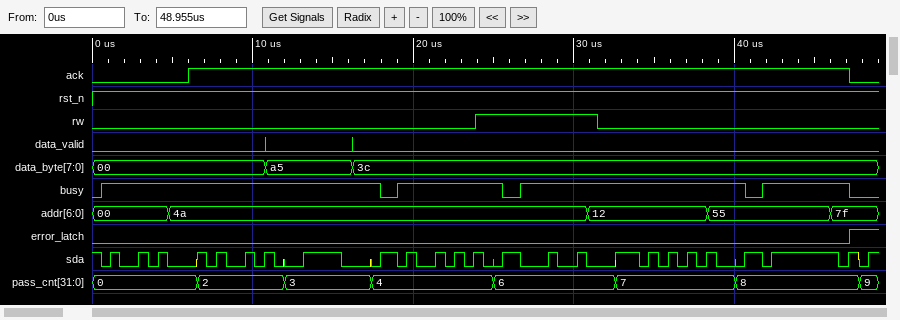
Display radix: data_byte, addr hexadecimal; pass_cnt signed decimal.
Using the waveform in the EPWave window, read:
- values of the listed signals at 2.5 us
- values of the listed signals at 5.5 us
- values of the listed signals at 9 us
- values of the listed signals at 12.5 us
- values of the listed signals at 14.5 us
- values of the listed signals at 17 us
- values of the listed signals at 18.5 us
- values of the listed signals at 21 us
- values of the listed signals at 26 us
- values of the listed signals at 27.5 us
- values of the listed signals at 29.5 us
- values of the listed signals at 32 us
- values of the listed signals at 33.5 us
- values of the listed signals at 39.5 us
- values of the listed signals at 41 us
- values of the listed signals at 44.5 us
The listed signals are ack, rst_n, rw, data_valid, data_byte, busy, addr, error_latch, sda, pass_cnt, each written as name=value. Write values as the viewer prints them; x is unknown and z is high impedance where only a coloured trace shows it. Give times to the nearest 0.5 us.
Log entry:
ack=0, rst_n=1, rw=0, data_valid=0, data_byte=00, busy=1, addr=00, error_latch=0, sda=0, pass_cnt=0
ack=0, rst_n=1, rw=0, data_valid=0, data_byte=00, busy=1, addr=4a, error_latch=0, sda=0, pass_cnt=0
ack=1, rst_n=1, rw=0, data_valid=0, data_byte=00, busy=1, addr=4a, error_latch=0, sda=0, pass_cnt=2
ack=1, rst_n=1, rw=0, data_valid=0, data_byte=a5, busy=1, addr=4a, error_latch=0, sda=0, pass_cnt=3
ack=1, rst_n=1, rw=0, data_valid=0, data_byte=a5, busy=1, addr=4a, error_latch=0, sda=1, pass_cnt=3
ack=1, rst_n=1, rw=0, data_valid=0, data_byte=3c, busy=1, addr=4a, error_latch=0, sda=0, pass_cnt=3
ack=1, rst_n=1, rw=0, data_valid=0, data_byte=3c, busy=0, addr=4a, error_latch=0, sda=1, pass_cnt=4
ack=1, rst_n=1, rw=0, data_valid=0, data_byte=3c, busy=1, addr=4a, error_latch=0, sda=0, pass_cnt=4
ack=1, rst_n=1, rw=1, data_valid=0, data_byte=3c, busy=0, addr=4a, error_latch=0, sda=1, pass_cnt=6
ack=1, rst_n=1, rw=1, data_valid=0, data_byte=3c, busy=1, addr=4a, error_latch=0, sda=0, pass_cnt=6
ack=1, rst_n=1, rw=1, data_valid=0, data_byte=3c, busy=1, addr=4a, error_latch=0, sda=0, pass_cnt=6
ack=1, rst_n=1, rw=0, data_valid=0, data_byte=3c, busy=1, addr=12, error_latch=0, sda=0, pass_cnt=6
ack=1, rst_n=1, rw=0, data_valid=0, data_byte=3c, busy=1, addr=12, error_latch=0, sda=1, pass_cnt=7
ack=1, rst_n=1, rw=0, data_valid=0, data_byte=3c, busy=1, addr=55, error_latch=0, sda=0, pass_cnt=7
ack=1, rst_n=1, rw=0, data_valid=0, data_byte=3c, busy=0, addr=55, error_latch=0, sda=1, pass_cnt=8
ack=1, rst_n=1, rw=0, data_valid=0, data_byte=3c, busy=1, addr=55, error_latch=0, sda=1, pass_cnt=8
